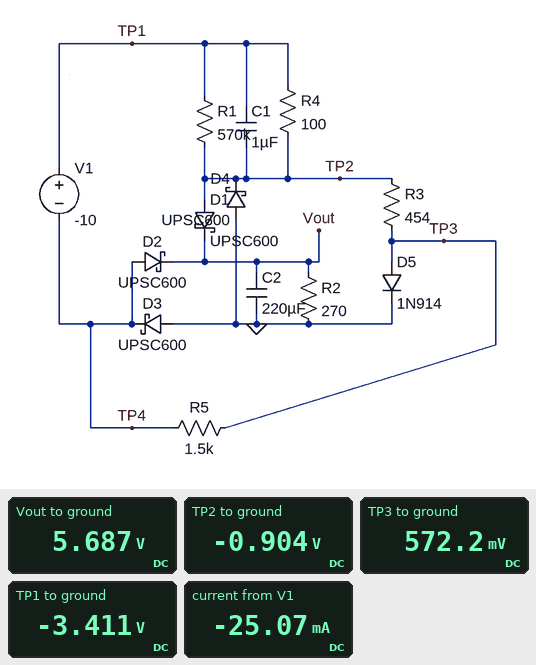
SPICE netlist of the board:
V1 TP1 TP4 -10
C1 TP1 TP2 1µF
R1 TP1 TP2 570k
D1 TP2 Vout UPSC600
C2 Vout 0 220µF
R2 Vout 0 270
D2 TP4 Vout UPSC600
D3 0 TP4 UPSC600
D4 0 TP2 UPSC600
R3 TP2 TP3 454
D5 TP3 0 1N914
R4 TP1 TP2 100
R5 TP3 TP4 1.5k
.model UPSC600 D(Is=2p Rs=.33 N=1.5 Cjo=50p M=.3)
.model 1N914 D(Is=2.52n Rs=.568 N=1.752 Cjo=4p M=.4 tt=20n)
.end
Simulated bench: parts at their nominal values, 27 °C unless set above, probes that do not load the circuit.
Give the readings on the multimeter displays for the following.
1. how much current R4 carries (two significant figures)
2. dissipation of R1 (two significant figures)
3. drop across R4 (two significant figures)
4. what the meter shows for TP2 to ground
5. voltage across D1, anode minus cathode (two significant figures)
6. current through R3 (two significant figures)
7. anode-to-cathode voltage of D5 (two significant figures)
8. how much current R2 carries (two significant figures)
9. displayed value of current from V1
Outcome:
25 mA
11 µW
2.5 V
-0.904 V
-6.6 V
3.3 mA
570 mV
21 mA
-25.07 mA
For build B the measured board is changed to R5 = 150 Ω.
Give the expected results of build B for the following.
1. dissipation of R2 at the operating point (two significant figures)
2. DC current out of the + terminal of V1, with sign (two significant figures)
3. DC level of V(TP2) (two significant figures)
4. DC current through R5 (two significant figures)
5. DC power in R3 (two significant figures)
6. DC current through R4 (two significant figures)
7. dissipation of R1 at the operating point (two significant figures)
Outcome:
58 mW
-42 mA
-930 mV
27 mA
6.2 mW
42 mA
31 µW
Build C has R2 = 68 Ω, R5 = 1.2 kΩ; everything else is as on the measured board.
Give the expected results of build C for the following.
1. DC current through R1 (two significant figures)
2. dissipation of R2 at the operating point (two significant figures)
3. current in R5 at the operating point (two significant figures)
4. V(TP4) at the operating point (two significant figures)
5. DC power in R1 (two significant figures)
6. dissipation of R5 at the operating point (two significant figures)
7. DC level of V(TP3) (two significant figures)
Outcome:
8.7 µA
150 mW
3.1 mA
4.1 V
43 µW
11 mW
430 mV
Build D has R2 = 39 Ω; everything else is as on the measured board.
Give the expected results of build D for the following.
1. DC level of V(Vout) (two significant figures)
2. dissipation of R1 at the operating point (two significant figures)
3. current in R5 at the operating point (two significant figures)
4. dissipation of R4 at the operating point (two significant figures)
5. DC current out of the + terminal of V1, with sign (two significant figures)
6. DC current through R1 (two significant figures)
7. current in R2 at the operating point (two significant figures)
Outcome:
2.2 V
61 µW
2.1 mA
350 mW
-59 mA
10 µA
57 mA
